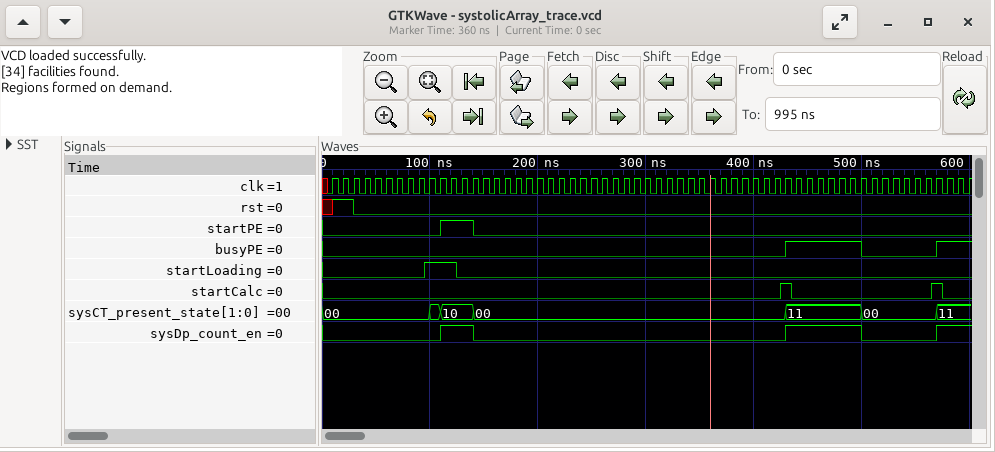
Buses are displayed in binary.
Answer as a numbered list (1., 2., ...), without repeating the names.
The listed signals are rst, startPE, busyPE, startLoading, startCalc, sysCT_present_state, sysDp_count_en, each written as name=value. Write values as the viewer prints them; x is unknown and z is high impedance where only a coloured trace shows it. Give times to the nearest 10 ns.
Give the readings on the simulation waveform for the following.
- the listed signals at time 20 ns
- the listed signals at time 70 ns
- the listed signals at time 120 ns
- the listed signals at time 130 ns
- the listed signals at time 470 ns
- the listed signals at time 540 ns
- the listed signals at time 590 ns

1. rst=1, startPE=0, busyPE=0, startLoading=0, startCalc=0, sysCT_present_state=00, sysDp_count_en=0
2. rst=0, startPE=0, busyPE=0, startLoading=0, startCalc=0, sysCT_present_state=00, sysDp_count_en=0
3. rst=0, startPE=1, busyPE=0, startLoading=1, startCalc=0, sysCT_present_state=10, sysDp_count_en=1
4. rst=0, startPE=1, busyPE=0, startLoading=0, startCalc=0, sysCT_present_state=10, sysDp_count_en=1
5. rst=0, startPE=0, busyPE=1, startLoading=0, startCalc=0, sysCT_present_state=11, sysDp_count_en=1
6. rst=0, startPE=0, busyPE=0, startLoading=0, startCalc=0, sysCT_present_state=00, sysDp_count_en=0
7. rst=0, startPE=0, busyPE=1, startLoading=0, startCalc=0, sysCT_present_state=11, sysDp_count_en=1
